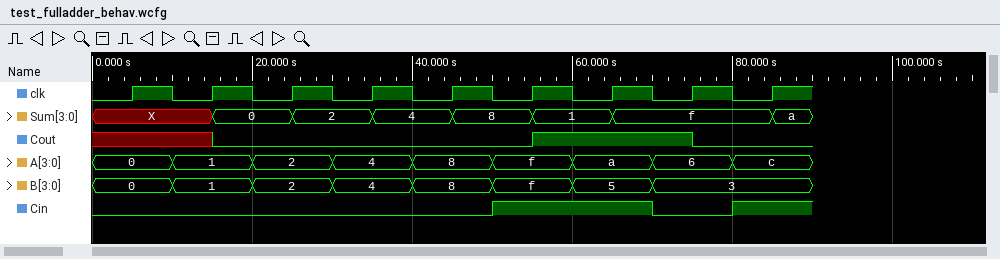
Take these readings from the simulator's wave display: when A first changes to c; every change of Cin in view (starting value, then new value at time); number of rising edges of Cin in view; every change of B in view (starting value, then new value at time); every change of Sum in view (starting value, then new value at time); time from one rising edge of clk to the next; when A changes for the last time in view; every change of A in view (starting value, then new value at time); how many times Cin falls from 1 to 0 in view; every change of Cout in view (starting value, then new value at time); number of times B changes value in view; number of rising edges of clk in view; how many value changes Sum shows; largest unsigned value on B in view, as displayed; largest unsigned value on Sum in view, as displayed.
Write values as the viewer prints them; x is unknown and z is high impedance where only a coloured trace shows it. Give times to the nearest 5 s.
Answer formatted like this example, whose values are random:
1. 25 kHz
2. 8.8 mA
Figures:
1. 80 s
2. 0, 1 at 50 s, 0 at 70 s, 1 at 80 s
3. 2
4. 0, 1 at 10 s, 2 at 20 s, 4 at 30 s, 8 at 40 s, f at 50 s, 5 at 60 s, 3 at 70 s
5. X, 0 at 15 s, 2 at 25 s, 4 at 35 s, 8 at 45 s, 1 at 55 s, f at 65 s, a at 85 s
6. 10 s
7. 80 s
8. 0, 1 at 10 s, 2 at 20 s, 4 at 30 s, 8 at 40 s, f at 50 s, a at 60 s, 6 at 70 s, c at 80 s
9. 1
10. x, 0 at 15 s, 1 at 55 s, 0 at 75 s
11. 7
12. 9
13. 7
14. f
15. f
